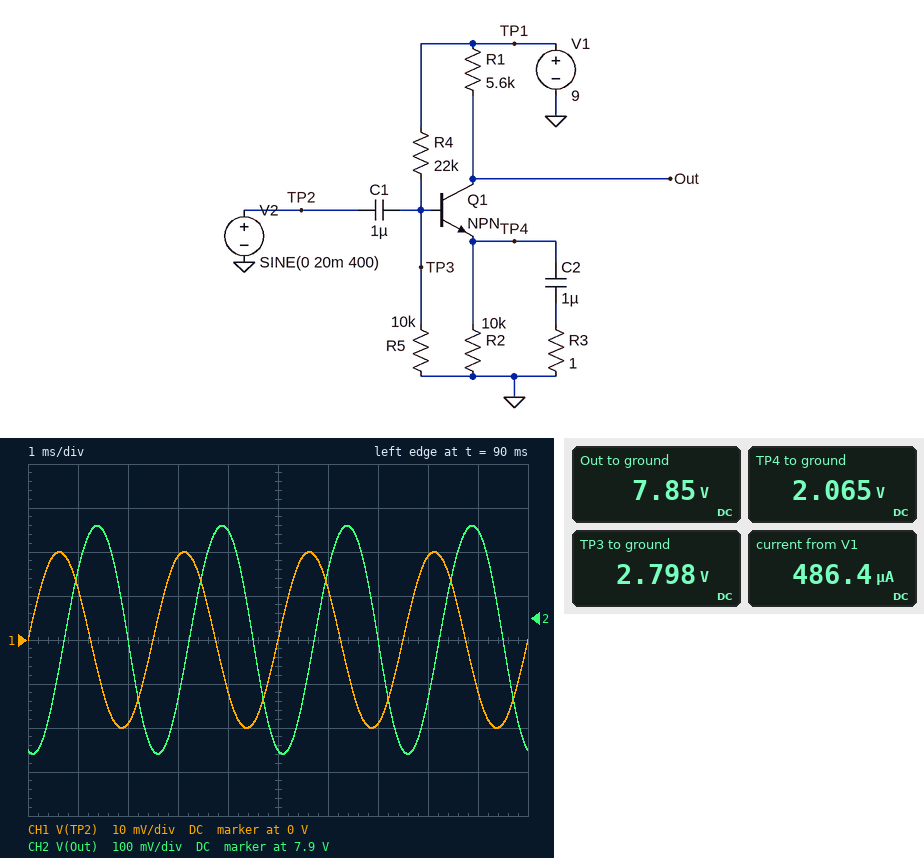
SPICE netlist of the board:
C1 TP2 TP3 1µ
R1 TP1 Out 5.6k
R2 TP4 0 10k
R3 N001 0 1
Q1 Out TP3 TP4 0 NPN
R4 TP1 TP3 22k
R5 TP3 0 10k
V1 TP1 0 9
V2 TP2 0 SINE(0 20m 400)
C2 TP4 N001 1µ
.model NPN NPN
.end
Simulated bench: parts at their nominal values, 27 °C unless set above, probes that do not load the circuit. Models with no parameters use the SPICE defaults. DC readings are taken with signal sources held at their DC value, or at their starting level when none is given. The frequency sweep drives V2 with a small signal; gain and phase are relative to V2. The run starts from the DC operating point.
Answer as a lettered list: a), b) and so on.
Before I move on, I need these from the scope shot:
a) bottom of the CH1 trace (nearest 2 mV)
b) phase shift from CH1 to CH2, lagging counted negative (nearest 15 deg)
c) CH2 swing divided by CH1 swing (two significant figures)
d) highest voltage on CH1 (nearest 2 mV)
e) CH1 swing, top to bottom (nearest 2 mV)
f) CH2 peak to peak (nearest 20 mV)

a) -20 mV
b) -105 deg
c) 13
d) 20 mV
e) 40 mV
f) 520 mV
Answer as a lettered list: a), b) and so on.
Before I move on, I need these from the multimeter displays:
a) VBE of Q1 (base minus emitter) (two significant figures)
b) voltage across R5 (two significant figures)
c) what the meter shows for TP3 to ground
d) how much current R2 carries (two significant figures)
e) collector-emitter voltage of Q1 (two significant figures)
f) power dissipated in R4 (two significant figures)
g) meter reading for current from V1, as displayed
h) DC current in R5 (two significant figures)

a) 730 mV
b) 2.8 V
c) 2.798 V
d) 210 µA
e) 5.8 V
f) 1.7 mW
g) 486.4 µA
h) 280 µA
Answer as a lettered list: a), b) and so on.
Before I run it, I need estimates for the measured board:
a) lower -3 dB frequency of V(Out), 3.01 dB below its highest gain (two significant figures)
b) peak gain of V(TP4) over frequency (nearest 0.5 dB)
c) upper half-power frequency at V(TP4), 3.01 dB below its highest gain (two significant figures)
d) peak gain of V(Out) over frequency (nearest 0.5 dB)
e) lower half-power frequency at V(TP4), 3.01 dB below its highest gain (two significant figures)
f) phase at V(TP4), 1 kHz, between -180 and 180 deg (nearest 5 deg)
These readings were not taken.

a) 1.3 kHz
b) -0.5 dB
c) 1.3 kHz
d) 33.0 dB
e) 22 Hz
f) -35 deg
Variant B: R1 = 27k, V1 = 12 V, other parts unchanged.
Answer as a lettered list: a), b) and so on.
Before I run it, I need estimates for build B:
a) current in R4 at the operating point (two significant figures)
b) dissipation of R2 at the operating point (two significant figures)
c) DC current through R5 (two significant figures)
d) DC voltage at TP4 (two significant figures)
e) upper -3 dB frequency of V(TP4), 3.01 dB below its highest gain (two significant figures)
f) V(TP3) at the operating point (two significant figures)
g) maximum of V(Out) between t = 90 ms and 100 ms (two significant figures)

a) 380 µA
b) 890 µW
c) 370 µA
d) 3.0 V
e) 1.9 kHz
f) 3.7 V
g) 5.3 V
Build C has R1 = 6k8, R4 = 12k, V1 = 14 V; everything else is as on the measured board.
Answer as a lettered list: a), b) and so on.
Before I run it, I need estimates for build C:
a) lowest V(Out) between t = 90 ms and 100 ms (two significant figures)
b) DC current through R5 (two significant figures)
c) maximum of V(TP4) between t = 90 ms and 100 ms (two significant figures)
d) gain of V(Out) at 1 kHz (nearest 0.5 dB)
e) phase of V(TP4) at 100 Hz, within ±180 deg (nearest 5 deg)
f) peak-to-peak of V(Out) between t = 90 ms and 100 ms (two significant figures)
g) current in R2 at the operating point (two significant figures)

a) 9.9 V
b) 630 µA
c) 5.6 V
d) 32.0 dB
e) 15 deg
f) 660 mV
g) 560 µA
